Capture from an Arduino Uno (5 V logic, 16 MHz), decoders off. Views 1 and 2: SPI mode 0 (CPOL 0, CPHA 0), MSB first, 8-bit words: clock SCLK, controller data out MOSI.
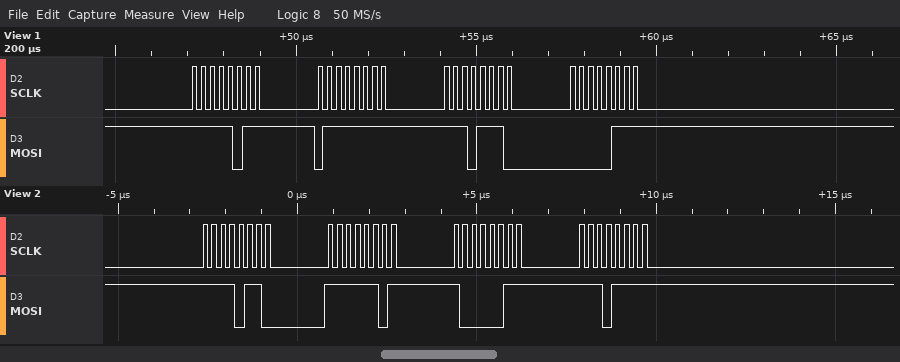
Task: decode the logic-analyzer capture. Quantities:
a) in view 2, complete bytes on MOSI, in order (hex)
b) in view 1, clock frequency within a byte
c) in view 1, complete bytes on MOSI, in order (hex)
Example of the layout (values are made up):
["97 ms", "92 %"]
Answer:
["F6 FD 83 EF", "4 MHz", "0xFB 0x7F 0xEE 0x07"]
